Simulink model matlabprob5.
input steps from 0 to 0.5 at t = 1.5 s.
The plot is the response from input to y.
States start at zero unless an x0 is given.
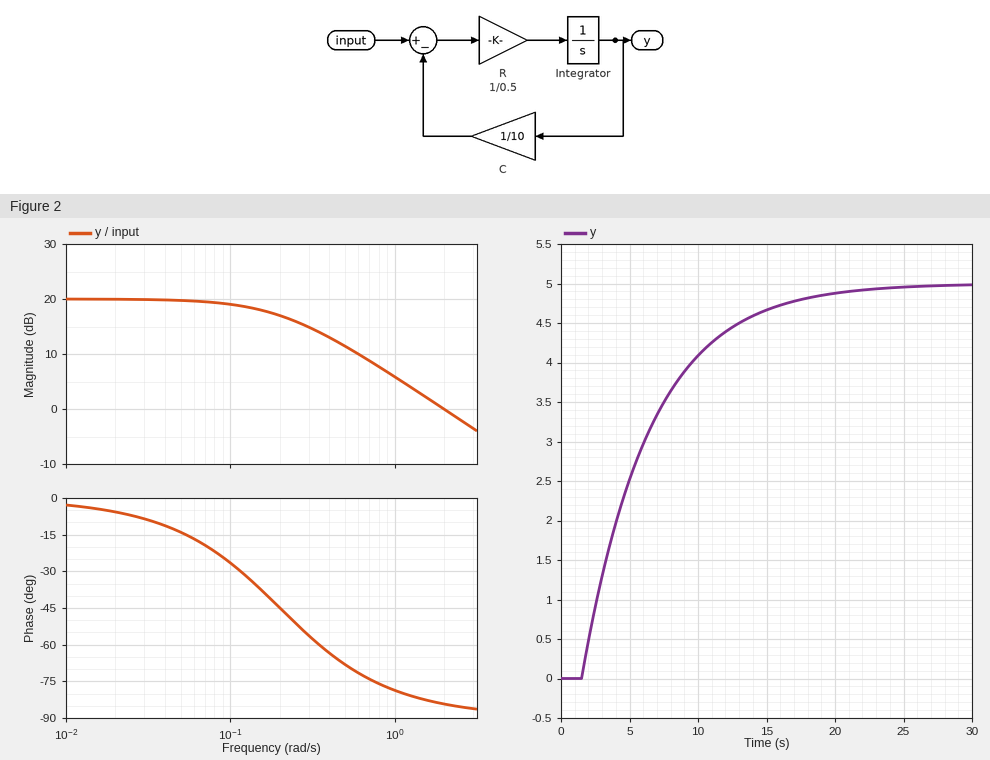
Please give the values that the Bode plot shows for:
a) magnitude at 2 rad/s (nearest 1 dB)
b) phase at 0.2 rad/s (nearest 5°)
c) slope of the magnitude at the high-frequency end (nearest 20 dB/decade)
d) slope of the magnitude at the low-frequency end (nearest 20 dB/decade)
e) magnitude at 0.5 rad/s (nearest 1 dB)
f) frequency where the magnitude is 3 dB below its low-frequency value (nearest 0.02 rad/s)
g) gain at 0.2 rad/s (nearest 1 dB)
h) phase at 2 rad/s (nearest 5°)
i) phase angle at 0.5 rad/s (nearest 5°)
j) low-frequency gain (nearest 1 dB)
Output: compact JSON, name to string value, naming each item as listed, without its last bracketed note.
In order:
{"magnitude at 2 rad/s": "0 dB", "phase at 0.2 rad/s": "-45°", "slope of the magnitude at the high-frequency end": "-20 dB/decade", "slope of the magnitude at the low-frequency end": "0 dB/decade", "magnitude at 0.5 rad/s": "11 dB", "frequency where the magnitude is 3 dB below its low-frequency value": "0.20 rad/s", "gain at 0.2 rad/s": "17 dB", "phase at 2 rad/s": "-85°", "phase angle at 0.5 rad/s": "-70°", "low-frequency gain": "20 dB"}
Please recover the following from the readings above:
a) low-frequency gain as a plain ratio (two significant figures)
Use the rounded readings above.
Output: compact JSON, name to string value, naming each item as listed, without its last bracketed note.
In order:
{"low-frequency gain as a plain ratio": "10"}
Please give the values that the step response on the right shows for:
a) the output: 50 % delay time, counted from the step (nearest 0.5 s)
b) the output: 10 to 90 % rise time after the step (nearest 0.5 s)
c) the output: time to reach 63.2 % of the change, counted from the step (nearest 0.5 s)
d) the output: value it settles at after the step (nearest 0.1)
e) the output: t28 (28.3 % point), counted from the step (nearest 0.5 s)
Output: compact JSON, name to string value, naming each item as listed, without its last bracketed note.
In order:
{"the output: 50 % delay time, counted from the step": "3.5 s", "the output: 10 to 90 % rise time after the step": "11.0 s", "the output: time to reach 63.2 % of the change, counted from the step": "5.0 s", "the output: value it settles at after the step": "5.0", "the output: t28 (28.3 % point), counted from the step": "1.5 s"}
